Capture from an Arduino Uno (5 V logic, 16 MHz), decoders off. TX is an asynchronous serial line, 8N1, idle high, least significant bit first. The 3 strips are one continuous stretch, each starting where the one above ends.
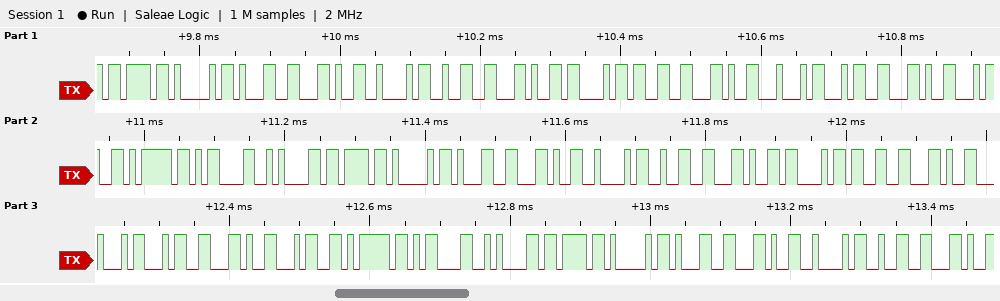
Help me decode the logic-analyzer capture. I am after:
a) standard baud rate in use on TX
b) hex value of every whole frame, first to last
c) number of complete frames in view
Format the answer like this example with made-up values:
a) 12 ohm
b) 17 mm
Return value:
a) 115200 baud
b) 7B 41 31 2C 42 32 2C 43 33 2C 44 34 2C 34 7D 0D 0A 7B 41 31 2C 42 32 2C 43 33 2C 44 34 2C 34 7D 0D 0A 7B 41 31 2C 42 32 2C
c) 41
